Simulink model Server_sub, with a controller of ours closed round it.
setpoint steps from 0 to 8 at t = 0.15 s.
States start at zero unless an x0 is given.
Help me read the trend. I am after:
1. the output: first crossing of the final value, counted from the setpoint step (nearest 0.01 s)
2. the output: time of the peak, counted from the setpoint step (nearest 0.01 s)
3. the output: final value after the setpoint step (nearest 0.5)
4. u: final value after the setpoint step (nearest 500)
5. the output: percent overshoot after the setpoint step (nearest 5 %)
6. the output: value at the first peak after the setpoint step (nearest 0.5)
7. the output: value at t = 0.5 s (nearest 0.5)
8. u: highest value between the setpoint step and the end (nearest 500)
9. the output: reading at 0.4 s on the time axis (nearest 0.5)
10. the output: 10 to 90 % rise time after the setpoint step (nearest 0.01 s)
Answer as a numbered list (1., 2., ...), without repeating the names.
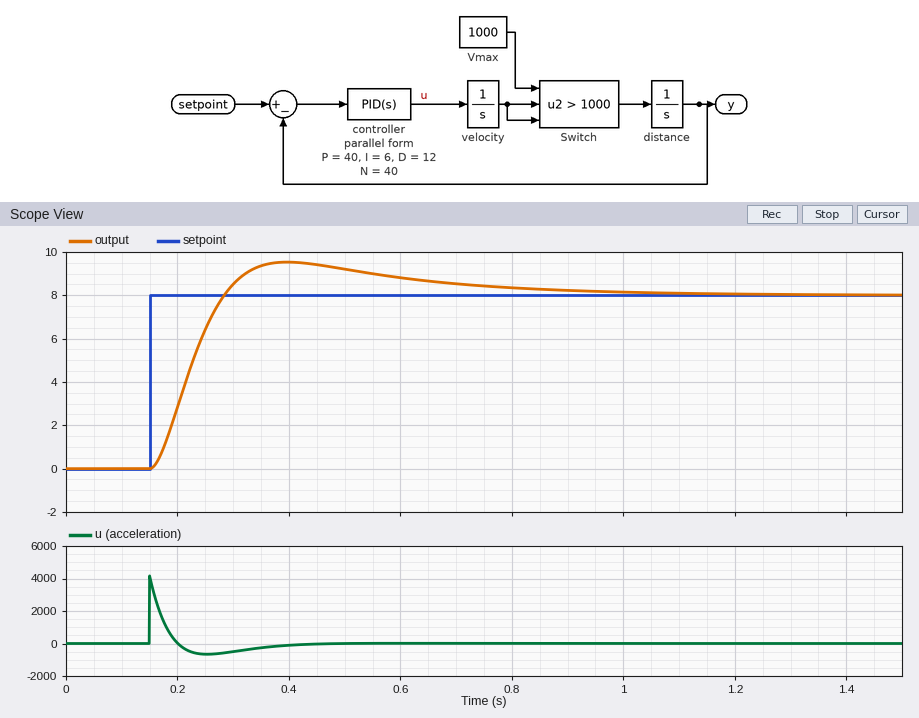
1. 0.13 s
2. 0.25 s
3. 8.0
4. 0
5. 20 %
6. 9.5
7. 9.0
8. 4000
9. 9.5
10. 0.09 s
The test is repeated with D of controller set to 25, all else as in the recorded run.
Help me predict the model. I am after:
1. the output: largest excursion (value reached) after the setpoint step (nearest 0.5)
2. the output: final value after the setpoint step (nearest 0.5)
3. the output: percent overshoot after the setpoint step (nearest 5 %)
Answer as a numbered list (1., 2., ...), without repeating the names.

1. 9.0
2. 8.0
3. 15 %
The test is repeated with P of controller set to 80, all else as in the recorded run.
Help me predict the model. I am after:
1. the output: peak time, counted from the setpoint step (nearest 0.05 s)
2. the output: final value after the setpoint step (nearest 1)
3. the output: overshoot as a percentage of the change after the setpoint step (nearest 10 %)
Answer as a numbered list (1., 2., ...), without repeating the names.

1. 0.20 s
2. 8
3. 30 %
